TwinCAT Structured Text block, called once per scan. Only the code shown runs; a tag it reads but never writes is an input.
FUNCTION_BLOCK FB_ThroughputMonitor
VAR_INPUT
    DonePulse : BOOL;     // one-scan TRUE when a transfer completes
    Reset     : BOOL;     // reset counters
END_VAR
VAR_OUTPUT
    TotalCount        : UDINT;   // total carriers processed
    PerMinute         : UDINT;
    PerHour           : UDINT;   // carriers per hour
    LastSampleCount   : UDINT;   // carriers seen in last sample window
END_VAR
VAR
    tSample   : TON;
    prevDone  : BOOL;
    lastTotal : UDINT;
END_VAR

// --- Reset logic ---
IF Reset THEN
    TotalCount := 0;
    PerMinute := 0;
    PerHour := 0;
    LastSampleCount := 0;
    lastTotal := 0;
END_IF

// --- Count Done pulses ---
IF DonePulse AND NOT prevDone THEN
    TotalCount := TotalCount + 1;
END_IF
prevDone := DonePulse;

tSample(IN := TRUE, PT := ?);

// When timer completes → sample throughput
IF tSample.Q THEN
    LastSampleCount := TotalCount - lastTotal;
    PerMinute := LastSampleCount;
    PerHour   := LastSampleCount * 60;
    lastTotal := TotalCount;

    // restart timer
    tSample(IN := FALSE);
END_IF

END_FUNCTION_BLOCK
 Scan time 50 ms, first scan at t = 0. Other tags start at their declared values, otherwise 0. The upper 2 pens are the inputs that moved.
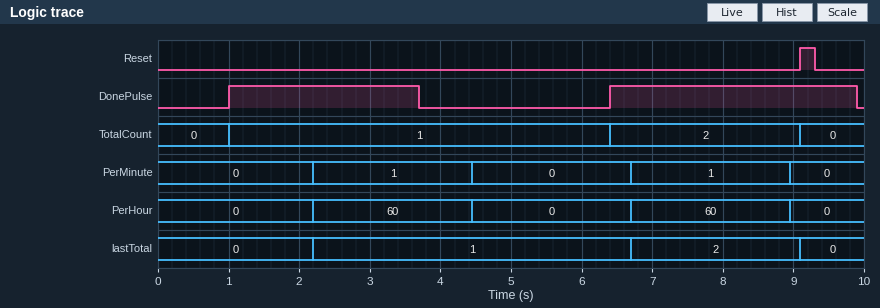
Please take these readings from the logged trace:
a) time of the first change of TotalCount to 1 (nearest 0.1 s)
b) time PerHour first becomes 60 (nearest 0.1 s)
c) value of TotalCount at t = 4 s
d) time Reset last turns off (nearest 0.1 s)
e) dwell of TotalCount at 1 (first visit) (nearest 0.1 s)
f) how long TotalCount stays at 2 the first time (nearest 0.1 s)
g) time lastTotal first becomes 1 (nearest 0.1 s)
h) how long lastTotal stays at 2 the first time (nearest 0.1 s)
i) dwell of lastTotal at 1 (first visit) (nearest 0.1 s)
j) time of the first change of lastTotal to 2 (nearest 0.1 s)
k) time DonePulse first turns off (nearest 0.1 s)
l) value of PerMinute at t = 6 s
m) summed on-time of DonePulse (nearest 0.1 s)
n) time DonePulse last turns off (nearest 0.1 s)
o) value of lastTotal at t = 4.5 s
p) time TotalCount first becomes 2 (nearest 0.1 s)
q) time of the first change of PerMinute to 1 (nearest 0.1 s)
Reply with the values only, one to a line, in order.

1.0 s
2.2 s
1
9.3 s
5.4 s
2.7 s
2.2 s
2.4 s
4.5 s
6.7 s
3.7 s
0
6.2 s
9.9 s
1
6.4 s
2.2 s
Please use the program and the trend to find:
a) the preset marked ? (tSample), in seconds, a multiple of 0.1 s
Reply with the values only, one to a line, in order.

2.2 s
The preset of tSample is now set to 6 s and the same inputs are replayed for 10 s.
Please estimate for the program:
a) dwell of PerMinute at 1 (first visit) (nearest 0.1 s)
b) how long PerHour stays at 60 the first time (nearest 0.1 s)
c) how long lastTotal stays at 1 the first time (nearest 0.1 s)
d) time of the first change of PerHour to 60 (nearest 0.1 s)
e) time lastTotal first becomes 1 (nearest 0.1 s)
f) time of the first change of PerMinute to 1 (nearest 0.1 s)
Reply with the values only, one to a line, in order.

3.1 s
3.1 s
3.1 s
6.0 s
6.0 s
6.0 s
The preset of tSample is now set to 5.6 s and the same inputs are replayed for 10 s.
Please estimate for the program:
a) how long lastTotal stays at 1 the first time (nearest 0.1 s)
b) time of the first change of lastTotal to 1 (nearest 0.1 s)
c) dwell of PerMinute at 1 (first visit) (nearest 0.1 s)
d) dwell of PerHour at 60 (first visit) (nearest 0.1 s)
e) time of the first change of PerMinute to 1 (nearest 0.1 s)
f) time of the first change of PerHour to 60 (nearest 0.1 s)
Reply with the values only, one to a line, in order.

3.5 s
5.6 s
3.5 s
3.5 s
5.6 s
5.6 s
